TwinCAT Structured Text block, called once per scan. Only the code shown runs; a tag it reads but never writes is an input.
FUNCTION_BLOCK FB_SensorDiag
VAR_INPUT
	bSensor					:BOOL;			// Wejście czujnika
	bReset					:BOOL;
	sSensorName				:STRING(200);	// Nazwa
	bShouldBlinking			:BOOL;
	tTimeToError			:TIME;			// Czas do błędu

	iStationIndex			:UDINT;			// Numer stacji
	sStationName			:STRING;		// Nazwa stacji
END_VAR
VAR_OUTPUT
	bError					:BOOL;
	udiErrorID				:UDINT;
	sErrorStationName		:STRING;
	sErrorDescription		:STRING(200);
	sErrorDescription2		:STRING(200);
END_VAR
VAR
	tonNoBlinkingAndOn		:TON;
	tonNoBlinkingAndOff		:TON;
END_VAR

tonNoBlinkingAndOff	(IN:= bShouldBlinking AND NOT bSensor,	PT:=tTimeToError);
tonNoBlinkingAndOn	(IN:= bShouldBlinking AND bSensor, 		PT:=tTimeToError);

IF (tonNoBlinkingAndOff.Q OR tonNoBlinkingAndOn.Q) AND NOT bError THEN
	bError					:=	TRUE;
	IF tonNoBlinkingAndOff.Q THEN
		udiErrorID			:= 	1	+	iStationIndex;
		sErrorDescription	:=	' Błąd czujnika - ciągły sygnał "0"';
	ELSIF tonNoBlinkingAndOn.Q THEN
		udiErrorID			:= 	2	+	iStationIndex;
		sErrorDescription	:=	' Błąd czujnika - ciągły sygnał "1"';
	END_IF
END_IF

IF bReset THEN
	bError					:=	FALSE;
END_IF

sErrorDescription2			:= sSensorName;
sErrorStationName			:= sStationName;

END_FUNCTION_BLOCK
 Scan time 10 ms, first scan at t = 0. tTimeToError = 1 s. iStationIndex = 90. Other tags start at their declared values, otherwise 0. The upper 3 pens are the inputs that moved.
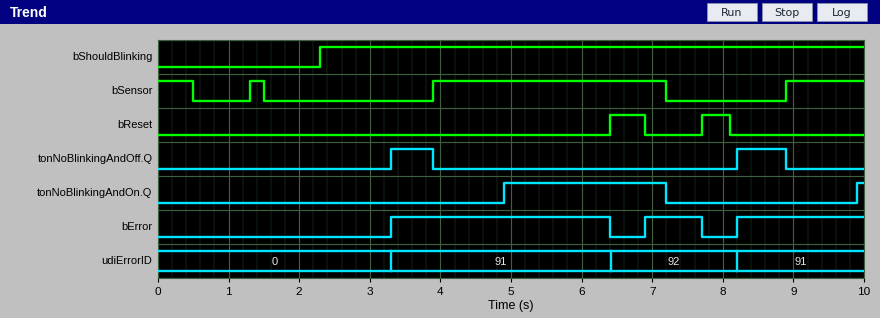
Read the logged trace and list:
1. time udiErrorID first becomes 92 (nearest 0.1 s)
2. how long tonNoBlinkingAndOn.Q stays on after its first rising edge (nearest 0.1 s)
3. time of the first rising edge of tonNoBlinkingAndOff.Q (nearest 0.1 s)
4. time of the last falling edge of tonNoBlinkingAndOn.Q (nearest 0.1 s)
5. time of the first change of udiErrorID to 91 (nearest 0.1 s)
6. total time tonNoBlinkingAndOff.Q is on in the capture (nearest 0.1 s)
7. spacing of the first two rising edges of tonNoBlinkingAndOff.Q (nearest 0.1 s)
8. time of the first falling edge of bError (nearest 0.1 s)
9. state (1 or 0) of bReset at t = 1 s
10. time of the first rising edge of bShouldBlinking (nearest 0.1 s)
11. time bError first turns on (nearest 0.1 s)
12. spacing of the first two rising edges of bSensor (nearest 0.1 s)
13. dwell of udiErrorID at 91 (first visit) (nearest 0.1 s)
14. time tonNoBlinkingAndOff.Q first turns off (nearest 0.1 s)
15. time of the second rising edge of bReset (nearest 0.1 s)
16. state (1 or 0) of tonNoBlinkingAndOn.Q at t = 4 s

6.4 s
2.3 s
3.3 s
7.2 s
3.3 s
1.3 s
4.9 s
6.4 s
0
2.3 s
3.3 s
2.6 s
3.1 s
3.9 s
7.7 s
0
